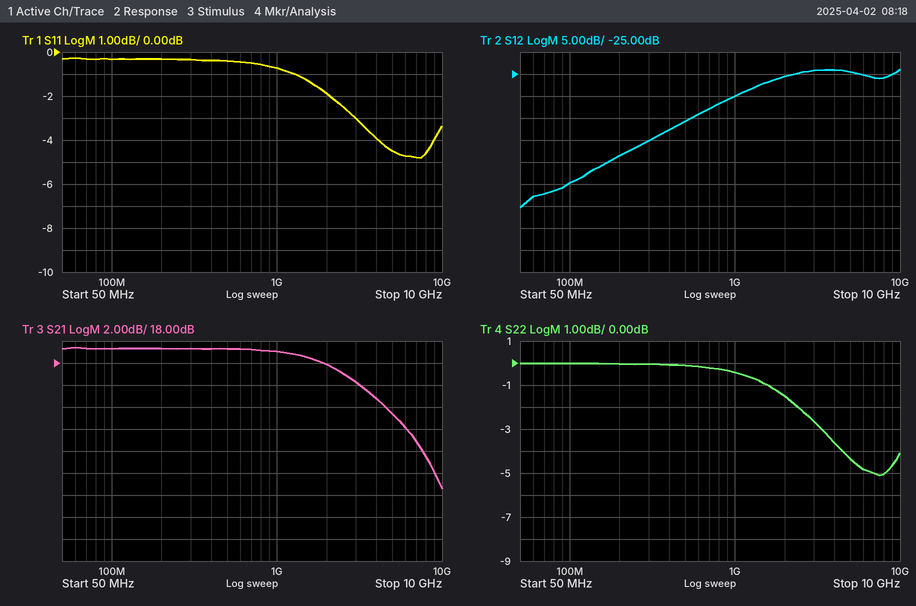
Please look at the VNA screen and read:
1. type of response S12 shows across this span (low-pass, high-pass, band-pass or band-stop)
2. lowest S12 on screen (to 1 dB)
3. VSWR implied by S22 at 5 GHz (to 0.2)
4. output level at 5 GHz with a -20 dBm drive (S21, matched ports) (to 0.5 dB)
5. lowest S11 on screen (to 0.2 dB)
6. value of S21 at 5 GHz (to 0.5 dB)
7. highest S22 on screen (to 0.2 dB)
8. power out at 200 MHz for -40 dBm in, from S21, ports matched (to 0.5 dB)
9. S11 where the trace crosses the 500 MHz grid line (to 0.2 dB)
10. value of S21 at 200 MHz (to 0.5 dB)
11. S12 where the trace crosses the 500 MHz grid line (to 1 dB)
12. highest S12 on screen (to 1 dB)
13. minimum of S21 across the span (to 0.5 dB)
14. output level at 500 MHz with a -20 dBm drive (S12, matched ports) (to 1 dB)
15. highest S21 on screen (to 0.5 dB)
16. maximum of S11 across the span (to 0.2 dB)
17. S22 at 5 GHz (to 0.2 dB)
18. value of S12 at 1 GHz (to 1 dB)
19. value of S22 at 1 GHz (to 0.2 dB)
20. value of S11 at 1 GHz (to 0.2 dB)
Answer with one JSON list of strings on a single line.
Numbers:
["high-pass", "-55 dB", "4.0", "-6.5 dBm", "-4.8 dB", "13.5 dB", "0.0 dB", "-20.5 dBm", "-0.4 dB", "19.5 dB", "-36 dB", "-24 dB", "6.5 dB", "-56 dBm", "19.5 dB", "-0.2 dB", "-4.4 dB", "-30 dB", "-0.4 dB", "-0.8 dB"]
